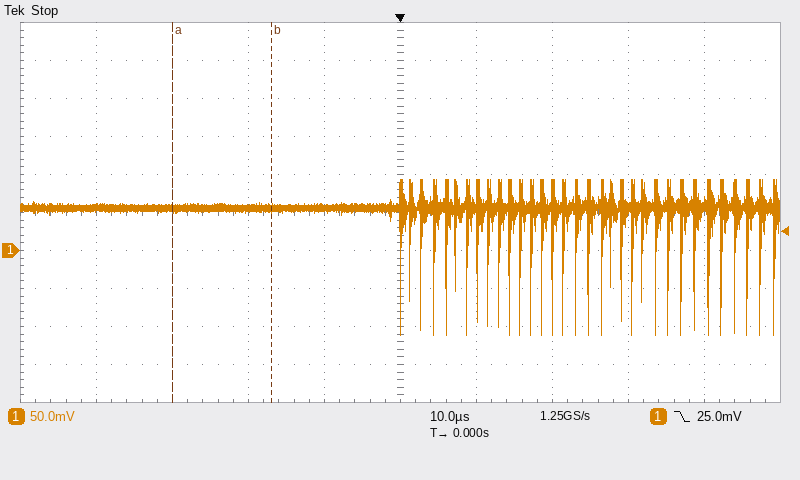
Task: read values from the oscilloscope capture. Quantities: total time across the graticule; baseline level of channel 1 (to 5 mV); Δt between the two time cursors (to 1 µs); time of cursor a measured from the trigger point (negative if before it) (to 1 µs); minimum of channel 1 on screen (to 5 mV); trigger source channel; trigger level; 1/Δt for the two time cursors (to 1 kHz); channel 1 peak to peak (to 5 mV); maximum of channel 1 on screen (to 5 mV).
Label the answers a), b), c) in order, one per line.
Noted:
a) 100 µs
b) 55 mV
c) 13 µs
d) -30 µs
e) -110 mV
f) channel 1
g) 25.0 mV
h) 77 kHz
i) 205 mV
j) 95 mV
